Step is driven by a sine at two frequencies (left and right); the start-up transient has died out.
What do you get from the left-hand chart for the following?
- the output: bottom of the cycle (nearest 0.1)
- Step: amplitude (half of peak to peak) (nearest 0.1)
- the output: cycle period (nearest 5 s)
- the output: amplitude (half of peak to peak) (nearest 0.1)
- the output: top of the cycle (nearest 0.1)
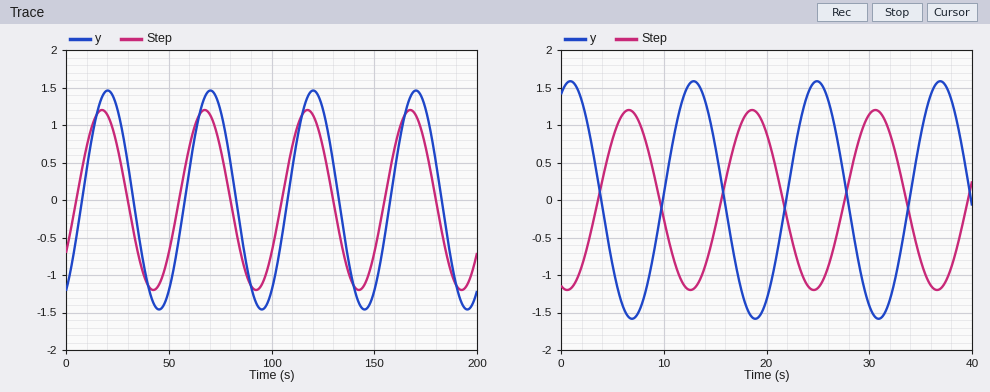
-1.5
1.2
50 s
1.5
1.5
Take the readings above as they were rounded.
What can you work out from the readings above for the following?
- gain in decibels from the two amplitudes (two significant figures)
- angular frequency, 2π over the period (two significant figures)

1.9 dB
0.13 rad/s
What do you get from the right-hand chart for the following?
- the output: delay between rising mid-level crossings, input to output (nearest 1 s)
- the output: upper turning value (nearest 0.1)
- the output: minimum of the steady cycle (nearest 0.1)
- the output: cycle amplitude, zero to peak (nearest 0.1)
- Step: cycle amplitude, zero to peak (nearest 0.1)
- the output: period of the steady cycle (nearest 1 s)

6 s
1.6
-1.6
1.6
1.2
12 s
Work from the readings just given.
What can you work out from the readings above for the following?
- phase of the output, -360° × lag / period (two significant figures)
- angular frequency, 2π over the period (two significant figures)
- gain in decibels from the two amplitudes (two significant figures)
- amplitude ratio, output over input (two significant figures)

-180°
0.52 rad/s
2.5 dB
1.3
